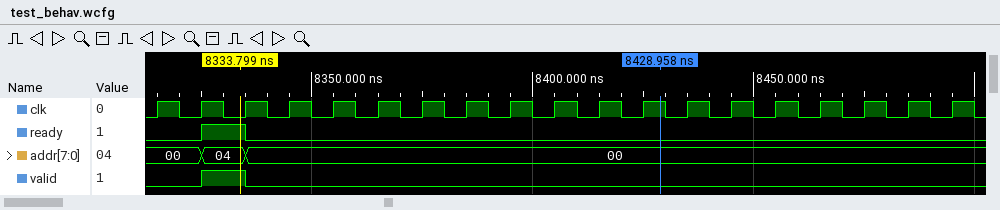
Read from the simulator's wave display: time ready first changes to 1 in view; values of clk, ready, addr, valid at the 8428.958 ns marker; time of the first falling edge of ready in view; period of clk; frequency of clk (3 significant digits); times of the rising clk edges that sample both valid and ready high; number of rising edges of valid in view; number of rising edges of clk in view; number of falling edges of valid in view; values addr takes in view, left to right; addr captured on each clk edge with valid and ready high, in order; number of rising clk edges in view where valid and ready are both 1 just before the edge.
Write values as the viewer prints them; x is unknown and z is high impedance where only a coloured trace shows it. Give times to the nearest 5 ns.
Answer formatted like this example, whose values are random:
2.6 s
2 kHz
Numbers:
8325 ns
clk=1, ready=0, addr=00, valid=0
8335 ns
10 ns
100 MHz
8335 ns
1
19
1
00, 04, 00
04
1
